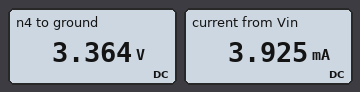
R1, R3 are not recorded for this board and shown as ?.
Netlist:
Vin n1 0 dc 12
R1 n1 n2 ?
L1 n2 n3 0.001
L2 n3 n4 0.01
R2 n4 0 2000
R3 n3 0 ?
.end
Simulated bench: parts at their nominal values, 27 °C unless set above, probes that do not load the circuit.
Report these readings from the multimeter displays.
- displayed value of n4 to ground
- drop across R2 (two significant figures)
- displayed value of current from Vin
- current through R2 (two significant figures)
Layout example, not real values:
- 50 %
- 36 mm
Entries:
- 3.364 V
- 3.4 V
- 3.925 mA
- 1.7 mA
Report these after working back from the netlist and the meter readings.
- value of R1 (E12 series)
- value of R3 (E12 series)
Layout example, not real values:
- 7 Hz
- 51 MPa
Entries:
- 2.2 kΩ
- 1.5 kΩ
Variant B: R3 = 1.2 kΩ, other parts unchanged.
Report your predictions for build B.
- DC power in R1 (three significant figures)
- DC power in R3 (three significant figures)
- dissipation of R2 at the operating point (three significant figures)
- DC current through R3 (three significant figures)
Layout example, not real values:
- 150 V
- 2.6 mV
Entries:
- 36.4 mW
- 7.76 mW
- 4.65 mW
- 2.54 mA
